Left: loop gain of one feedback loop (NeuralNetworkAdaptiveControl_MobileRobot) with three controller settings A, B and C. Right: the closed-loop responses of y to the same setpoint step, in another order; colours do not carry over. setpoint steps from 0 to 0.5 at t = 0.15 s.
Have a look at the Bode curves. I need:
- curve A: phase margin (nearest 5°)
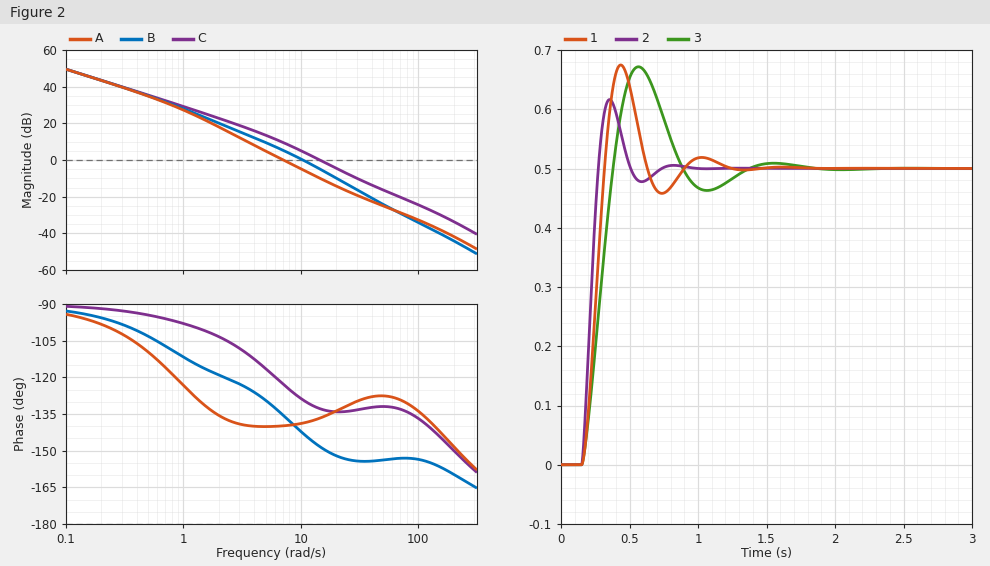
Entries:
40°
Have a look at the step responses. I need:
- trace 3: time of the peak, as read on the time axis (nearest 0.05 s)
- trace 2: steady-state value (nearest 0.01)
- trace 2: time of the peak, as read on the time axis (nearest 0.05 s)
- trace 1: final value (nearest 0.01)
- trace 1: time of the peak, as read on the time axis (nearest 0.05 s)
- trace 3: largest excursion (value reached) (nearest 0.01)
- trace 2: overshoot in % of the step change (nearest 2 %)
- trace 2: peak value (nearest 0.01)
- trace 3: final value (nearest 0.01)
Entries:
0.55 s
0.50
0.35 s
0.50
0.45 s
0.67
24 %
0.62
0.50
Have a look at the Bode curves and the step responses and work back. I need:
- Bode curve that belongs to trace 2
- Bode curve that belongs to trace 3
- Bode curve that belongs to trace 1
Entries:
C
A
B
